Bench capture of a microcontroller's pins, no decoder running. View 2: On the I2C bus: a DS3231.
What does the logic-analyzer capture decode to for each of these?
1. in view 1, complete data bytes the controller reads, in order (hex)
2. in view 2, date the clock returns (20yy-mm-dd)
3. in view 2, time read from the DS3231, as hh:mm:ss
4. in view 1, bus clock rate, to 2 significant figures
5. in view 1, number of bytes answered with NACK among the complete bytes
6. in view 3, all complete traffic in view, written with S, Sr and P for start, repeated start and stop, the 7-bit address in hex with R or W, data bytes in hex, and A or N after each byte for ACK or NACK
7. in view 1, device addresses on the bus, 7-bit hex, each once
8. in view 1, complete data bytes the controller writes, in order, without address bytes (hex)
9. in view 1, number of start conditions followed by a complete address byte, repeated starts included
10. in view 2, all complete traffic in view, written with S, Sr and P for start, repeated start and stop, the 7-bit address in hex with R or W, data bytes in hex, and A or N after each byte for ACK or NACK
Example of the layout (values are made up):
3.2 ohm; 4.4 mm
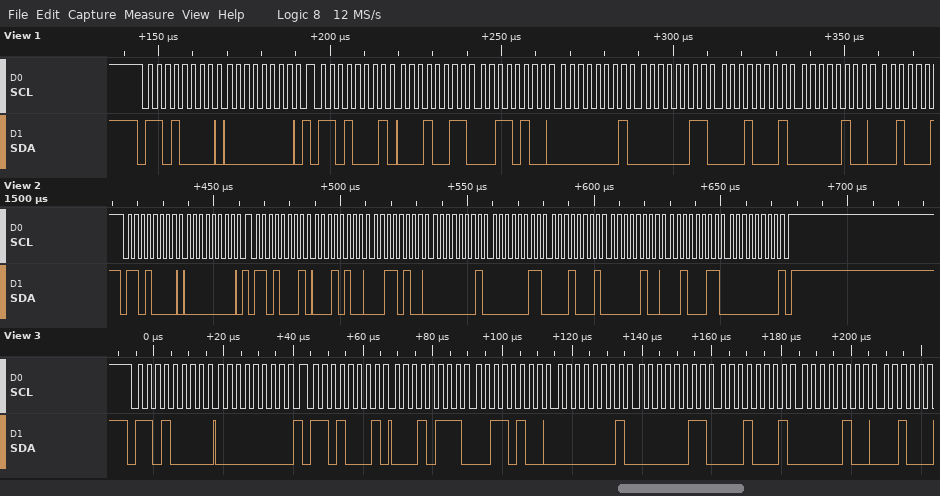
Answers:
13 34 01 03 11 04; 2023-04-11; 01:34:14; 400 kHz; 0; S 68W A 00 A Sr 68R A 17 A 34 A 01 A 03 A 11 A 04 A; 0x68; 00; 2; S 68W A 00 A Sr 68R A 14 A 34 A 01 A 03 A 11 A 04 A 23 A 00 N P
